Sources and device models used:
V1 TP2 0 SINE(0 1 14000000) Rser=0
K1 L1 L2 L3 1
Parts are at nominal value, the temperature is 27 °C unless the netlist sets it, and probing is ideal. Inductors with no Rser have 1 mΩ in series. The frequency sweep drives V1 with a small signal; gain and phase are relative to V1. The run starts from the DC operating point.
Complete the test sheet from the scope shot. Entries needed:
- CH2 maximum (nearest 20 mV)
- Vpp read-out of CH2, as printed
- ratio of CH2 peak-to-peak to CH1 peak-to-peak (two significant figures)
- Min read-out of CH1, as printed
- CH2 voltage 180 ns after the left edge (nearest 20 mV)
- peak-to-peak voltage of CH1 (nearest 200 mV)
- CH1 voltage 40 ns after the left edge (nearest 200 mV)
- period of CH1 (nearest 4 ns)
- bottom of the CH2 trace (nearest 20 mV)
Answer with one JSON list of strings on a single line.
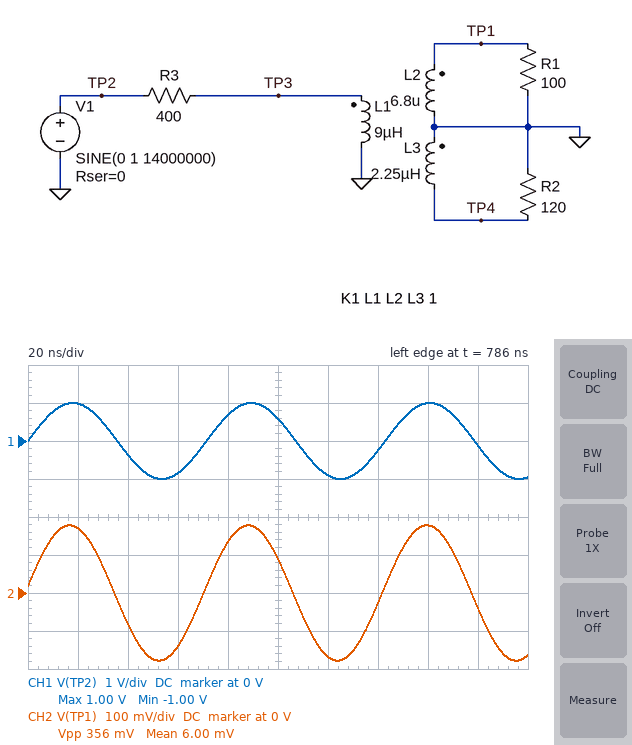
["180 mV", "356 mV", "0.18", "-1.00 V", "-40 mV", "2.0 V", "-400 mV", "72 ns", "-180 mV"]
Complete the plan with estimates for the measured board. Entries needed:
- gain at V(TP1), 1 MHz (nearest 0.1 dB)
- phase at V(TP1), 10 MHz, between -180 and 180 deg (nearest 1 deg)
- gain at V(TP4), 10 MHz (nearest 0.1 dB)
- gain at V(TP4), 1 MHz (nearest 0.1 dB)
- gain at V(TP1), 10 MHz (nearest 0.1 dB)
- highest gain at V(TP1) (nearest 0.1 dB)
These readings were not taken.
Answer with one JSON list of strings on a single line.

["-19.9 dB", "8 deg", "-19.8 dB", "-24.7 dB", "-15.0 dB", "-14.9 dB"]
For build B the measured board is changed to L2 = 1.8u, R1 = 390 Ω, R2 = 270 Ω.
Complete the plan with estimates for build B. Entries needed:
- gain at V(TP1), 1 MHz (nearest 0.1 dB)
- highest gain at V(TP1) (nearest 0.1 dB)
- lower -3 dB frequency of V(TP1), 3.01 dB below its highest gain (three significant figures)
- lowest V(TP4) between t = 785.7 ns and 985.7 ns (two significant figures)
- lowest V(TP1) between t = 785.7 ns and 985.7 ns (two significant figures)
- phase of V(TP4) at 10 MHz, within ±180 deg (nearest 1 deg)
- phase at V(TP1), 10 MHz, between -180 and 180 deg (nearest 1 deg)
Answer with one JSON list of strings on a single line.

["-24.2 dB", "-10.9 dB", "4.49 MHz", "-300 mV", "-270 mV", "-156 deg", "24 deg"]
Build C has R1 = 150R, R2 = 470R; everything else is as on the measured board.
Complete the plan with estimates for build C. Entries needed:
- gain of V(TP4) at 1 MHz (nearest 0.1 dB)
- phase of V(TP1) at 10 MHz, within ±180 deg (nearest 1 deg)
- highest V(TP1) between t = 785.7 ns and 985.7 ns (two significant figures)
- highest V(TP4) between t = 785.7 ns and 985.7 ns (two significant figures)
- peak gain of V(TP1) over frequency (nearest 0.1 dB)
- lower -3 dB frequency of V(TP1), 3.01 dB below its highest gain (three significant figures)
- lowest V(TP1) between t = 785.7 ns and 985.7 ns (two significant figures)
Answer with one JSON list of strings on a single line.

["-23.8 dB", "12 deg", "270 mV", "150 mV", "-11.4 dB", "2.19 MHz", "-270 mV"]
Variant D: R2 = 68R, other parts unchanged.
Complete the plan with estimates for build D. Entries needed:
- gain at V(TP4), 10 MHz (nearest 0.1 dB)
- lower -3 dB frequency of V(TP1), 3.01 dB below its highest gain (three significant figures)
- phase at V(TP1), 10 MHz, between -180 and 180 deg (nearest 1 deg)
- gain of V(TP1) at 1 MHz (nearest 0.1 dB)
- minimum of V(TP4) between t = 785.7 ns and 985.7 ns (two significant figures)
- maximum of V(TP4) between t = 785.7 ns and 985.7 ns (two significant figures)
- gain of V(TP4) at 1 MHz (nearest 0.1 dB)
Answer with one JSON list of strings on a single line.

["-20.9 dB", "1.29 MHz", "7 deg", "-20.3 dB", "-91 mV", "91 mV", "-25.1 dB"]
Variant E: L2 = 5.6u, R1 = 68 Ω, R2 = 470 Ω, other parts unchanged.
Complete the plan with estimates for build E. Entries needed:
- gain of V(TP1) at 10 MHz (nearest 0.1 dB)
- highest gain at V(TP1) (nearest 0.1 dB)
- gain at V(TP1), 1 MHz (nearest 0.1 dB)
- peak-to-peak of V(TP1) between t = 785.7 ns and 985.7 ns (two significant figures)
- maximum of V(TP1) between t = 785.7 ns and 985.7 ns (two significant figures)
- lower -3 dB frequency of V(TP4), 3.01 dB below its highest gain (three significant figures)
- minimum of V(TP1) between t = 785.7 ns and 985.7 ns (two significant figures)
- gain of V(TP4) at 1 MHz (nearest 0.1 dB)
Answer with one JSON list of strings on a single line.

["-15.9 dB", "-15.8 dB", "-20.7 dB", "320 mV", "160 mV", "1.45 MHz", "-160 mV", "-24.7 dB"]
